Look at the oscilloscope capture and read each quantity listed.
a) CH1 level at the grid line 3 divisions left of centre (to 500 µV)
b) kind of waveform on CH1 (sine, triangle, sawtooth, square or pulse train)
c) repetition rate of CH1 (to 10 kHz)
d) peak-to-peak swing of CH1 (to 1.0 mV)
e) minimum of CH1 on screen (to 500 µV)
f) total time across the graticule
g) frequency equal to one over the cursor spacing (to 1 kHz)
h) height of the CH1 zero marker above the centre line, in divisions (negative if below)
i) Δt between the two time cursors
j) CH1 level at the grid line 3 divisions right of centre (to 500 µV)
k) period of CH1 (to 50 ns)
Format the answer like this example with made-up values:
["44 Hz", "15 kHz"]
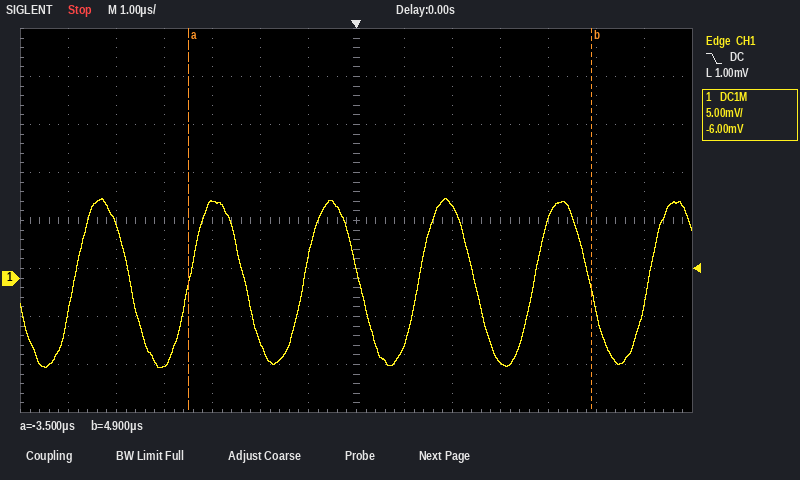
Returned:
["8.0 mV", "sine", "420 kHz", "18.0 mV", "-9.5 mV", "14 µs", "119 kHz", "-1.2 div", "8.4 µs", "-9.0 mV", "2.40 µs"]
